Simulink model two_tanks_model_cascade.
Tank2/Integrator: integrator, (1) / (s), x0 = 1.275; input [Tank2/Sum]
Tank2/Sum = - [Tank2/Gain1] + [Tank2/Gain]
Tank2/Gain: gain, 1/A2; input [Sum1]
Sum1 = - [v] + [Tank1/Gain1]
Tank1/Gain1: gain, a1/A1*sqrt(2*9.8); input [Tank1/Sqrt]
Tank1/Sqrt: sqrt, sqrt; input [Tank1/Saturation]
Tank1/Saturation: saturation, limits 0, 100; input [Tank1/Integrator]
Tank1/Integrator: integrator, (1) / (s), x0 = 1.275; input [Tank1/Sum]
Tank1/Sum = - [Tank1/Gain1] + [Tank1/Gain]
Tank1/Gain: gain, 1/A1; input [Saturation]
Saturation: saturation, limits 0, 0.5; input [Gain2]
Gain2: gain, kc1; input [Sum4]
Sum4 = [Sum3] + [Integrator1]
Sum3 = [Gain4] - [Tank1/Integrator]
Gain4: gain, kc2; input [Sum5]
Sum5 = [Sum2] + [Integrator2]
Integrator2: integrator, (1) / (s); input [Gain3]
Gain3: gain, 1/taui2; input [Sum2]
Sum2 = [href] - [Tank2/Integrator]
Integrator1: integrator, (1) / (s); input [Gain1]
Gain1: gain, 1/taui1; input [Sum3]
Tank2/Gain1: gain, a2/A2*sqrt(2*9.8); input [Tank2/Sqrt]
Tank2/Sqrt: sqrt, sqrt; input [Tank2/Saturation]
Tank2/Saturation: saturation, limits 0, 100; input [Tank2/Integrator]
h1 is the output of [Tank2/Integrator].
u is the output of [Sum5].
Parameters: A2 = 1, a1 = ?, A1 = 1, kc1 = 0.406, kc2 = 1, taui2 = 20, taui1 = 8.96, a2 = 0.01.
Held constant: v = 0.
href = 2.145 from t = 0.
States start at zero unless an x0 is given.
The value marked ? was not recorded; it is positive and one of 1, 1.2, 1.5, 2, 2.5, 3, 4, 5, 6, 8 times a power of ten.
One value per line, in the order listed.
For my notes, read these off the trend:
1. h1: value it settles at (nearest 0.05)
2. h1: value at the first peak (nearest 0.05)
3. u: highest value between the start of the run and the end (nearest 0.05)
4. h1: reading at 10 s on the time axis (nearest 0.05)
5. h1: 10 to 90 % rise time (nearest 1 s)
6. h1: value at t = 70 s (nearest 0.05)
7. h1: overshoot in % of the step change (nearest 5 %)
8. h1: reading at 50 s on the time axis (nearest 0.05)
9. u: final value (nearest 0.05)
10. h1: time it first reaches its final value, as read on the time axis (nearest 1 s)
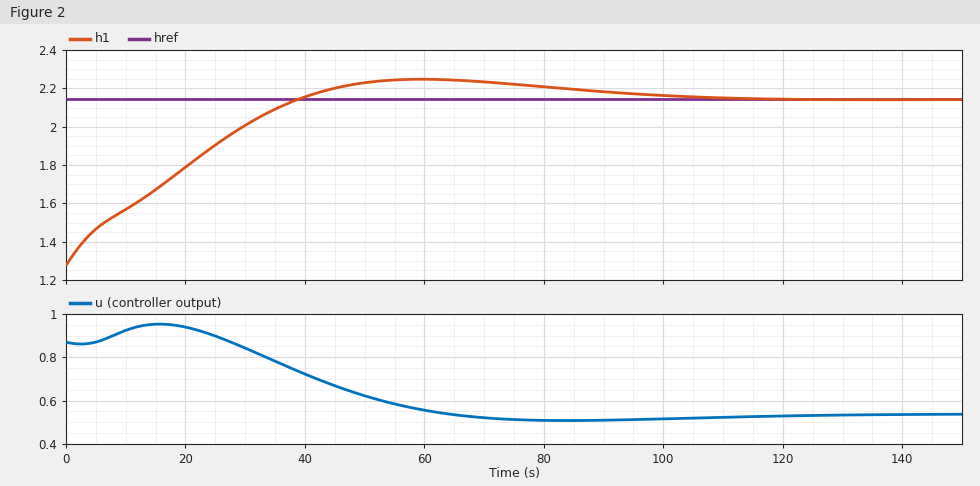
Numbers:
2.15
2.25
0.95
1.55
31 s
2.25
10 %
2.25
0.55
39 s
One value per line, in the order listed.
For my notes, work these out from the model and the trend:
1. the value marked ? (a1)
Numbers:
0.02
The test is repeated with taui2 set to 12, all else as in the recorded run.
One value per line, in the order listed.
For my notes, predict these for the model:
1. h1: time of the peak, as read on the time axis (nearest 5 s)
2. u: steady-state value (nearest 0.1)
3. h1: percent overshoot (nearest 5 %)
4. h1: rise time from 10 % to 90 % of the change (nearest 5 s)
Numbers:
45 s
0.5
25 %
25 s
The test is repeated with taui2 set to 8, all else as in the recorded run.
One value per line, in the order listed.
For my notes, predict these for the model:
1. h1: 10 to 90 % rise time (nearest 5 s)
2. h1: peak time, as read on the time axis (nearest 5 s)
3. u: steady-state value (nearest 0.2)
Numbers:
20 s
40 s
0.6
